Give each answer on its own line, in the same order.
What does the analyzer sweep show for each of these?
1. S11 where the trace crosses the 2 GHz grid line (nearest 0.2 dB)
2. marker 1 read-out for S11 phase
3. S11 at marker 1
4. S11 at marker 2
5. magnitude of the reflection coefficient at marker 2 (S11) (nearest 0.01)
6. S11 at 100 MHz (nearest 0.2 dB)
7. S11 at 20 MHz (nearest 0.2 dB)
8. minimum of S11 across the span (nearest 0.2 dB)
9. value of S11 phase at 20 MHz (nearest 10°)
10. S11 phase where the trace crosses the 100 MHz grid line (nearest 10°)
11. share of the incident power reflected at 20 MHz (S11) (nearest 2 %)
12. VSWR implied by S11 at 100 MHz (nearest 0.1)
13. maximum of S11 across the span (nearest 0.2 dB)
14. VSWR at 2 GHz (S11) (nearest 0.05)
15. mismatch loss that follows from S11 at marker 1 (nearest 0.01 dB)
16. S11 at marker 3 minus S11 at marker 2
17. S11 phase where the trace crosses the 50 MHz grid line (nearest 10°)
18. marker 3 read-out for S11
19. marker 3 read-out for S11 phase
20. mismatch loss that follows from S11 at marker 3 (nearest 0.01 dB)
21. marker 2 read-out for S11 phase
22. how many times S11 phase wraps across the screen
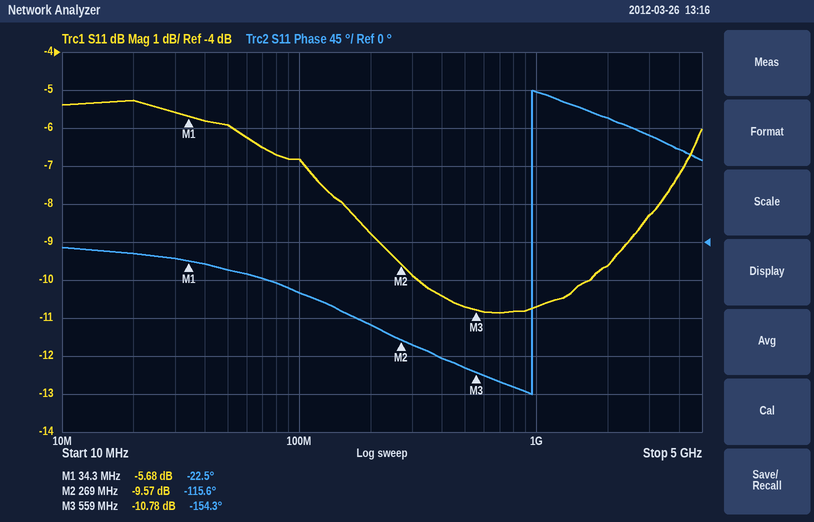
-9.6 dB
-22.5°
-5.68 dB
-9.57 dB
0.33
-6.8 dB
-5.2 dB
-10.8 dB
-10°
-60°
30 %
2.7
-5.2 dB
2.00
1.37 dB
-1.21 dB
-30°
-10.78 dB
-154.3°
0.38 dB
-115.6°
1
